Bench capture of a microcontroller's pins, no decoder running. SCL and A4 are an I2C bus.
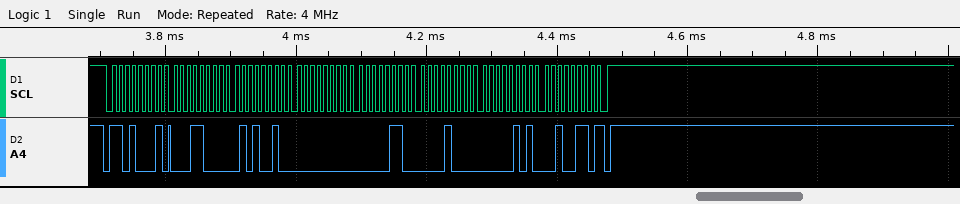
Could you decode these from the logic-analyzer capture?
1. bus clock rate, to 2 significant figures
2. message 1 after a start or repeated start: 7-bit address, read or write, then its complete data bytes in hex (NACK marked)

100 kHz
0x68 read: 18 52 00 06 08 05 26 NACK
